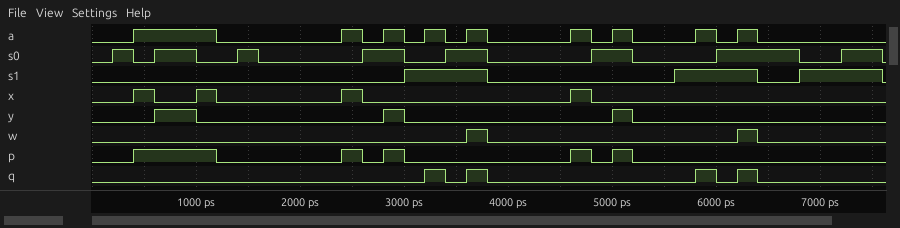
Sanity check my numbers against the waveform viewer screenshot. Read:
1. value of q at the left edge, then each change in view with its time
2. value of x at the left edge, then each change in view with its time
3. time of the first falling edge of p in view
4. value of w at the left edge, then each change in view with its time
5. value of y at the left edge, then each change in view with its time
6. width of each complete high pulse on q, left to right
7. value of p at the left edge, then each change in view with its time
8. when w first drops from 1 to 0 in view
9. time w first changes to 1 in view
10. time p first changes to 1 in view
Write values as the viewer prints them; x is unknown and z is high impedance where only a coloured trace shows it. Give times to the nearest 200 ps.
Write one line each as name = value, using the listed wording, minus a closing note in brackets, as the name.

value of q at the left edge, then each change in view with its time = 0, 1 at 3200 ps, 0 at 3400 ps, 1 at 3600 ps, 0 at 3800 ps, 1 at 5800 ps, 0 at 6000 ps, 1 at 6200 ps, 0 at 6400 ps
value of x at the left edge, then each change in view with its time = 0, 1 at 400 ps, 0 at 600 ps, 1 at 1000 ps, 0 at 1200 ps, 1 at 2400 ps, 0 at 2600 ps, 1 at 4600 ps, 0 at 4800 ps
time of the first falling edge of p in view = 1200 ps
value of w at the left edge, then each change in view with its time = 0, 1 at 3600 ps, 0 at 3800 ps, 1 at 6200 ps, 0 at 6400 ps
value of y at the left edge, then each change in view with its time = 0, 1 at 600 ps, 0 at 1000 ps, 1 at 2800 ps, 0 at 3000 ps, 1 at 5000 ps, 0 at 5200 ps
width of each complete high pulse on q, left to right = 200 ps, 200 ps, 200 ps, 200 ps
value of p at the left edge, then each change in view with its time = 0, 1 at 400 ps, 0 at 1200 ps, 1 at 2400 ps, 0 at 2600 ps, 1 at 2800 ps, 0 at 3000 ps, 1 at 4600 ps, 0 at 4800 ps, 1 at 5000 ps, 0 at 5200 ps
when w first drops from 1 to 0 in view = 3800 ps
time w first changes to 1 in view = 3600 ps
time p first changes to 1 in view = 400 ps
